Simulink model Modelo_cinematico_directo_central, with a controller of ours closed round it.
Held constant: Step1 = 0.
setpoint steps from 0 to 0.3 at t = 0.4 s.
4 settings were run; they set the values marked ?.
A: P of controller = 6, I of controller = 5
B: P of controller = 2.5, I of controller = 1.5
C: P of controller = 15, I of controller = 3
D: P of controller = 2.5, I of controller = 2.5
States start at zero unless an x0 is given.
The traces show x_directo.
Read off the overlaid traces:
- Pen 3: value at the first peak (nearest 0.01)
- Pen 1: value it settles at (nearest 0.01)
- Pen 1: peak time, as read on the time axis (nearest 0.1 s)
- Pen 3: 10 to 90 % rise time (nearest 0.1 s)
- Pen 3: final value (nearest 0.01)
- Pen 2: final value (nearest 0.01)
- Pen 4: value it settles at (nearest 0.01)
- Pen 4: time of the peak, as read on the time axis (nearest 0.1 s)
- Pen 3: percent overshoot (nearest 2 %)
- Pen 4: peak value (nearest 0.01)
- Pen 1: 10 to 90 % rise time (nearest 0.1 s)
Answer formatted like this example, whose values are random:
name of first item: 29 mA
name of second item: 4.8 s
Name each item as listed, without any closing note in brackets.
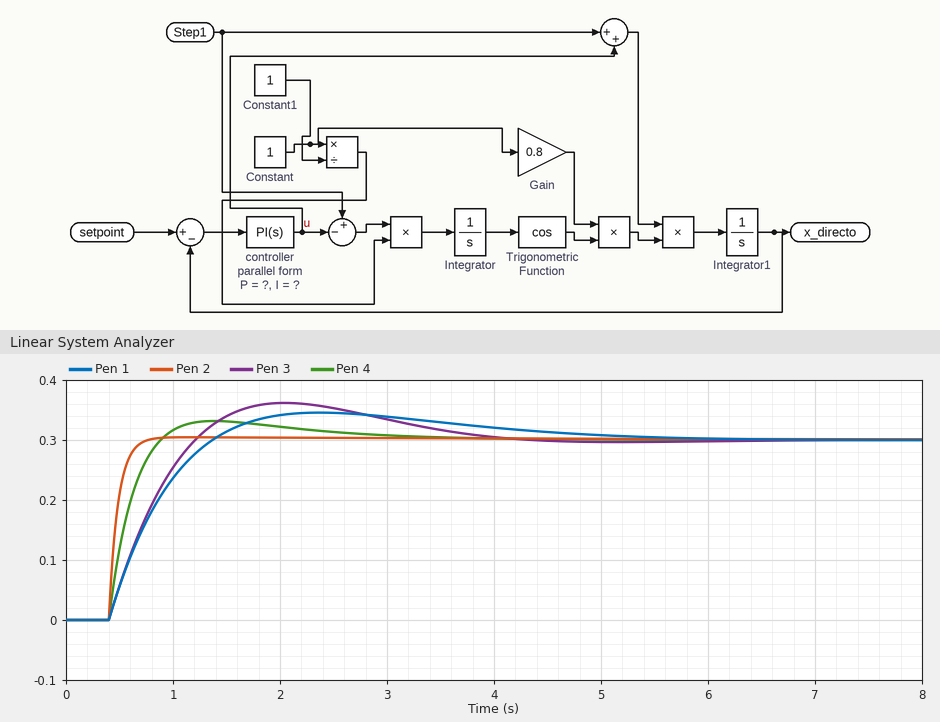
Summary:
Pen 3: value at the first peak: 0.36
Pen 1: value it settles at: 0.30
Pen 1: peak time, as read on the time axis: 2.4 s
Pen 3: 10 to 90 % rise time: 0.6 s
Pen 3: final value: 0.30
Pen 2: final value: 0.30
Pen 4: value it settles at: 0.30
Pen 4: time of the peak, as read on the time axis: 1.4 s
Pen 3: percent overshoot: 20 %
Pen 4: peak value: 0.33
Pen 1: 10 to 90 % rise time: 0.7 s
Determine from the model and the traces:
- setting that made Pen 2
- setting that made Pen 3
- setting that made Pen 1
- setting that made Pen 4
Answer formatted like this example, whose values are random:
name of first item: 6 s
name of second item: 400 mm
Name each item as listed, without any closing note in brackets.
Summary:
setting that made Pen 2: C
setting that made Pen 3: D
setting that made Pen 1: B
setting that made Pen 4: A
